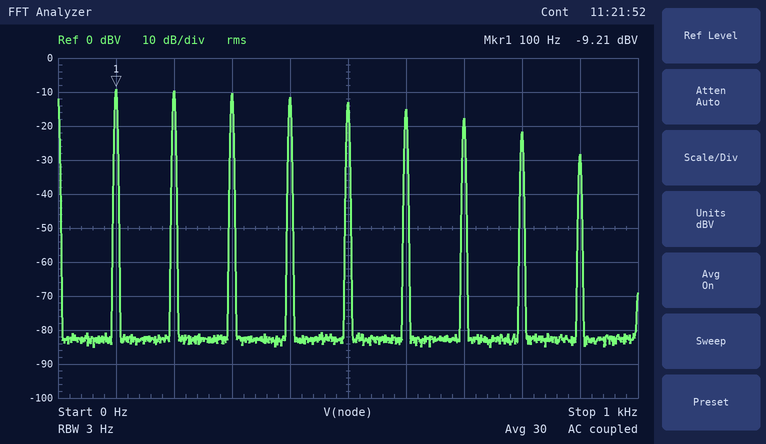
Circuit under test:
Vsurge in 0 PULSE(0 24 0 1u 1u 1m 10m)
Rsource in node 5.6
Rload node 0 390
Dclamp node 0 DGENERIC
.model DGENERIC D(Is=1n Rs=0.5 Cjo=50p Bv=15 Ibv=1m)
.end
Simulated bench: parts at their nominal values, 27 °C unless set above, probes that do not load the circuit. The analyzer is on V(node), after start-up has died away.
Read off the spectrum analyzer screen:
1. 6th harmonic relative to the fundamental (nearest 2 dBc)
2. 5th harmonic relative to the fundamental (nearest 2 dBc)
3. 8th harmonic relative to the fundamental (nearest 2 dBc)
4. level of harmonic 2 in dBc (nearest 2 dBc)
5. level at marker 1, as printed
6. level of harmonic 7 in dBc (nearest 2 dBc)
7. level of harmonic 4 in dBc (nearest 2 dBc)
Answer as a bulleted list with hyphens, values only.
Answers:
- -6 dBc
- -4 dBc
- -12 dBc
- 0 dBc
- -9.21 dBV
- -8 dBc
- -2 dBc
